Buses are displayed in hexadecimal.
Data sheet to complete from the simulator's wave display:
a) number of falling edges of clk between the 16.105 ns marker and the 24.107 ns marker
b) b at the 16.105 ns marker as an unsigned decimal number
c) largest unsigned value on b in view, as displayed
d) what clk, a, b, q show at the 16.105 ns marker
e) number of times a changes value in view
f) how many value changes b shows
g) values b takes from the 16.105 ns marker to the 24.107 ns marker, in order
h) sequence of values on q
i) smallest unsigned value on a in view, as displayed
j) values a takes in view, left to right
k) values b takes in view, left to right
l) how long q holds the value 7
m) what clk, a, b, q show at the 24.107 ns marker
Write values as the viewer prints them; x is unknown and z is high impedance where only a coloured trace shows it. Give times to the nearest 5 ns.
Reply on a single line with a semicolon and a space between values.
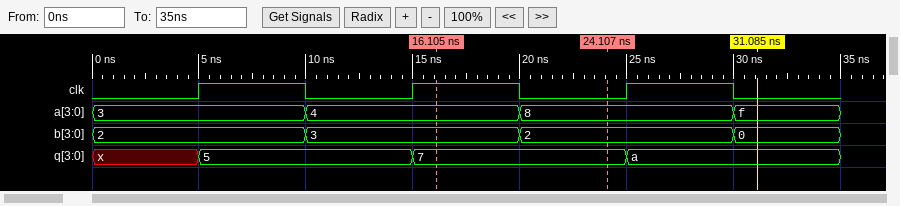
1; 3; 3; clk=1, a=4, b=3, q=7; 3; 3; 3, 2; x, 5, 7, a; 3; 3, 4, 8, f; 2, 3, 2, 0; 10 ns; clk=0, a=8, b=2, q=7
